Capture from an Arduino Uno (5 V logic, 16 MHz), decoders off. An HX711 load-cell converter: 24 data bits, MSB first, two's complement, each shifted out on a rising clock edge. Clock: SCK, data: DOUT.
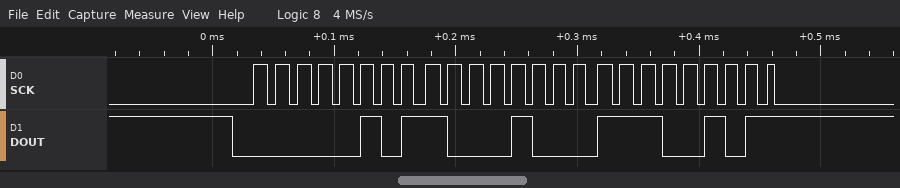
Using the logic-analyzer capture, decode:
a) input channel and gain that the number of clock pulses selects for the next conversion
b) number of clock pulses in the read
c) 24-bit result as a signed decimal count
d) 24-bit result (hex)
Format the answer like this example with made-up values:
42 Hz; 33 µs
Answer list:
channel A, gain 128; 25; 362725; 0x0588E5
